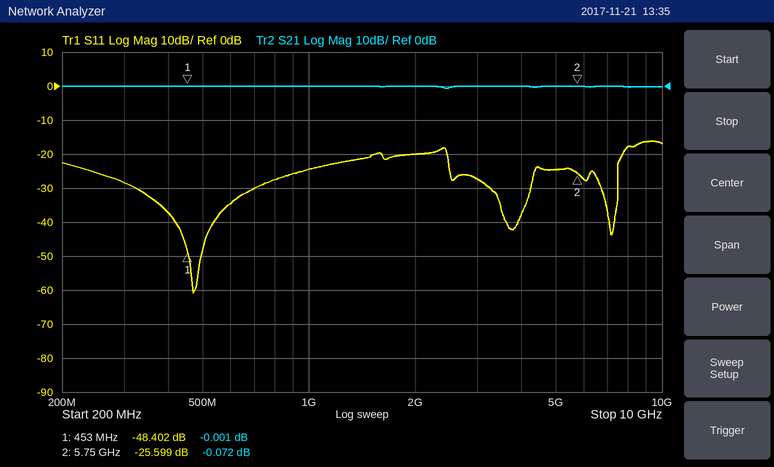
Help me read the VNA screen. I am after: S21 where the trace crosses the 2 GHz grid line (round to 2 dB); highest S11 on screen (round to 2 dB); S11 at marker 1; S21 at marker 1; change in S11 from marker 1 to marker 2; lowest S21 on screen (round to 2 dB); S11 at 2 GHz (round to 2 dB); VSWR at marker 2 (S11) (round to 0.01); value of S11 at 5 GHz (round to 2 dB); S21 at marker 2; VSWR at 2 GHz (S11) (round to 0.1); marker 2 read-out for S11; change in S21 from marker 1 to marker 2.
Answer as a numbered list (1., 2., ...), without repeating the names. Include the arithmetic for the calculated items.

1. 0 dB
2. -16 dB
3. -48.402 dB
4. -0.001 dB
5. -25.599 − (-48.402) = 22.803 dB
6. 0 dB
7. -20 dB
8. (1 + 0.0525)/(1 − 0.0525) ≈ 1.11
9. -24 dB
10. -0.072 dB
11. |Γ| = 10^(-20/20) = 0.1000; VSWR = (1 + 0.1000)/(1 − 0.1000) ≈ 1.2
12. -25.599 dB
13. -0.072 − (-0.001) = -0.071 dB
